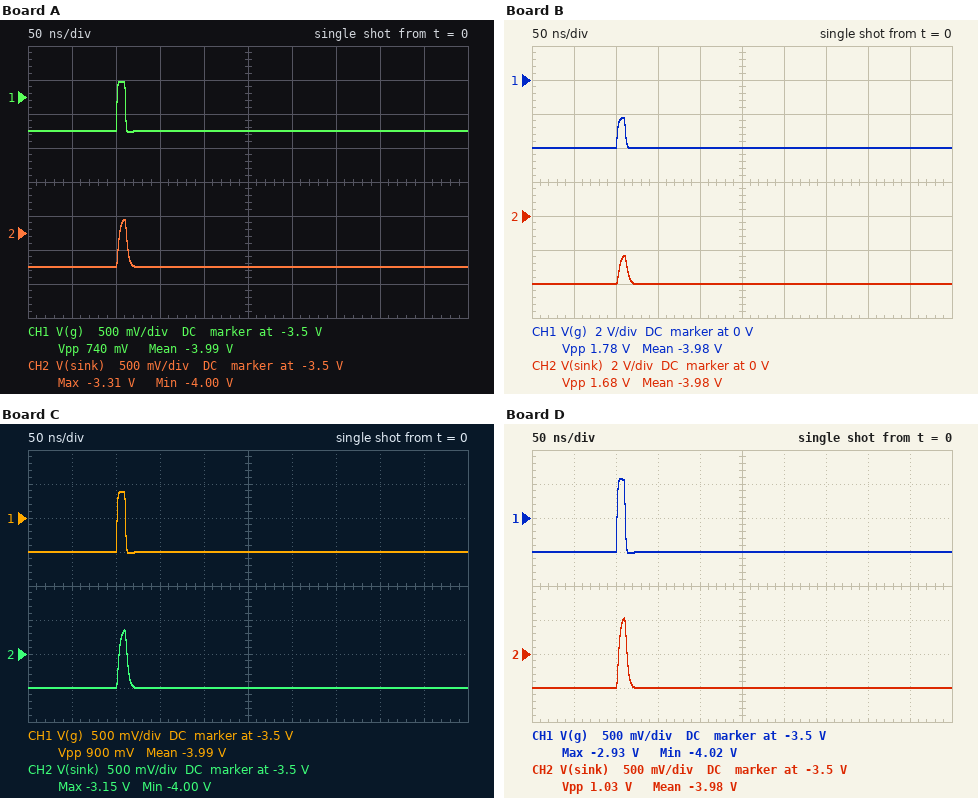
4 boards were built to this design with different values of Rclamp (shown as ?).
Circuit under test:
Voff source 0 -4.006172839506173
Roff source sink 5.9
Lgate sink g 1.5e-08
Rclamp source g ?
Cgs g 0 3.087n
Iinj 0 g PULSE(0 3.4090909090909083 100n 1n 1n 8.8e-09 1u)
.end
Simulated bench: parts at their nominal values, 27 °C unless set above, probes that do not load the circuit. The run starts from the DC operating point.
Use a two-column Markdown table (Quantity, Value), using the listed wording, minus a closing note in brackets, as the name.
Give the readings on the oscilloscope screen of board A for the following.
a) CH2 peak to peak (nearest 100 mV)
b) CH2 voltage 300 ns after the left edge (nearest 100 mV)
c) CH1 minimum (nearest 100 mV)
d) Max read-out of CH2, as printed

| Quantity | Value |
|---|---|
| CH2 peak to peak | 700 mV |
| CH2 voltage 300 ns after the left edge | -4.0 V |
| CH1 minimum | -4.0 V |
| Max read-out of CH2, as printed | -3.31 V |
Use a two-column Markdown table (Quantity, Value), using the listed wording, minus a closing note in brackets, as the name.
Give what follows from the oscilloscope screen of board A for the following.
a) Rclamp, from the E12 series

| Quantity | Value |
|---|---|
| Rclamp, from the E12 series | 0.22 Ω |
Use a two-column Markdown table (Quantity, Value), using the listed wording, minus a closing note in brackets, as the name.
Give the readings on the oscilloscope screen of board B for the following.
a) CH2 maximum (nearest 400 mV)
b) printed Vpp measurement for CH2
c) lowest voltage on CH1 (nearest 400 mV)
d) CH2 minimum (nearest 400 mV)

| Quantity | Value |
|---|---|
| CH2 maximum | -2.4 V |
| printed Vpp measurement for CH2 | 1.68 V |
| lowest voltage on CH1 | -4.0 V |
| CH2 minimum | -4.0 V |
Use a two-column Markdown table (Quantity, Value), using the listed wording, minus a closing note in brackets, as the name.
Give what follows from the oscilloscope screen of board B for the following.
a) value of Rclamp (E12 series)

| Quantity | Value |
|---|---|
| value of Rclamp | 0.56 Ω |
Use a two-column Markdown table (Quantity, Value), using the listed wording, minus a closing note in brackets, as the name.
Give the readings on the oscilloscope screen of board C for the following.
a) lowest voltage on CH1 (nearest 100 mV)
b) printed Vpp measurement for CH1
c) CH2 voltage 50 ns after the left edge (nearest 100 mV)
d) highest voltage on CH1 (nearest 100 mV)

| Quantity | Value |
|---|---|
| lowest voltage on CH1 | -4.0 V |
| printed Vpp measurement for CH1 | 900 mV |
| CH2 voltage 50 ns after the left edge | -4.0 V |
| highest voltage on CH1 | -3.1 V |
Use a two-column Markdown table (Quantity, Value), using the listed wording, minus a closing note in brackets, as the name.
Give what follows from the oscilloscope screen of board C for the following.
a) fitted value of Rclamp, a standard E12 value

| Quantity | Value |
|---|---|
| fitted value of Rclamp, a standard E12 value | 0.27 Ω |
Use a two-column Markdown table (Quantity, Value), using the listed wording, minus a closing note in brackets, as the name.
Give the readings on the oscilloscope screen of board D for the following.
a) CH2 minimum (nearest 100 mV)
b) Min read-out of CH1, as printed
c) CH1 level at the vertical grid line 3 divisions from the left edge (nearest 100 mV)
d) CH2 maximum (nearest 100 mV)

| Quantity | Value |
|---|---|
| CH2 minimum | -4.0 V |
| Min read-out of CH1, as printed | -4.02 V |
| CH1 level at the vertical grid line 3 divisions from the left edge | -4.0 V |
| CH2 maximum | -3.0 V |
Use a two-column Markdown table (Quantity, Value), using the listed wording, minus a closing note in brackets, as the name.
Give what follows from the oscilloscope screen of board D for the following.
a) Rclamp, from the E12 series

| Quantity | Value |
|---|---|
| Rclamp, from the E12 series | 0.33 Ω |
